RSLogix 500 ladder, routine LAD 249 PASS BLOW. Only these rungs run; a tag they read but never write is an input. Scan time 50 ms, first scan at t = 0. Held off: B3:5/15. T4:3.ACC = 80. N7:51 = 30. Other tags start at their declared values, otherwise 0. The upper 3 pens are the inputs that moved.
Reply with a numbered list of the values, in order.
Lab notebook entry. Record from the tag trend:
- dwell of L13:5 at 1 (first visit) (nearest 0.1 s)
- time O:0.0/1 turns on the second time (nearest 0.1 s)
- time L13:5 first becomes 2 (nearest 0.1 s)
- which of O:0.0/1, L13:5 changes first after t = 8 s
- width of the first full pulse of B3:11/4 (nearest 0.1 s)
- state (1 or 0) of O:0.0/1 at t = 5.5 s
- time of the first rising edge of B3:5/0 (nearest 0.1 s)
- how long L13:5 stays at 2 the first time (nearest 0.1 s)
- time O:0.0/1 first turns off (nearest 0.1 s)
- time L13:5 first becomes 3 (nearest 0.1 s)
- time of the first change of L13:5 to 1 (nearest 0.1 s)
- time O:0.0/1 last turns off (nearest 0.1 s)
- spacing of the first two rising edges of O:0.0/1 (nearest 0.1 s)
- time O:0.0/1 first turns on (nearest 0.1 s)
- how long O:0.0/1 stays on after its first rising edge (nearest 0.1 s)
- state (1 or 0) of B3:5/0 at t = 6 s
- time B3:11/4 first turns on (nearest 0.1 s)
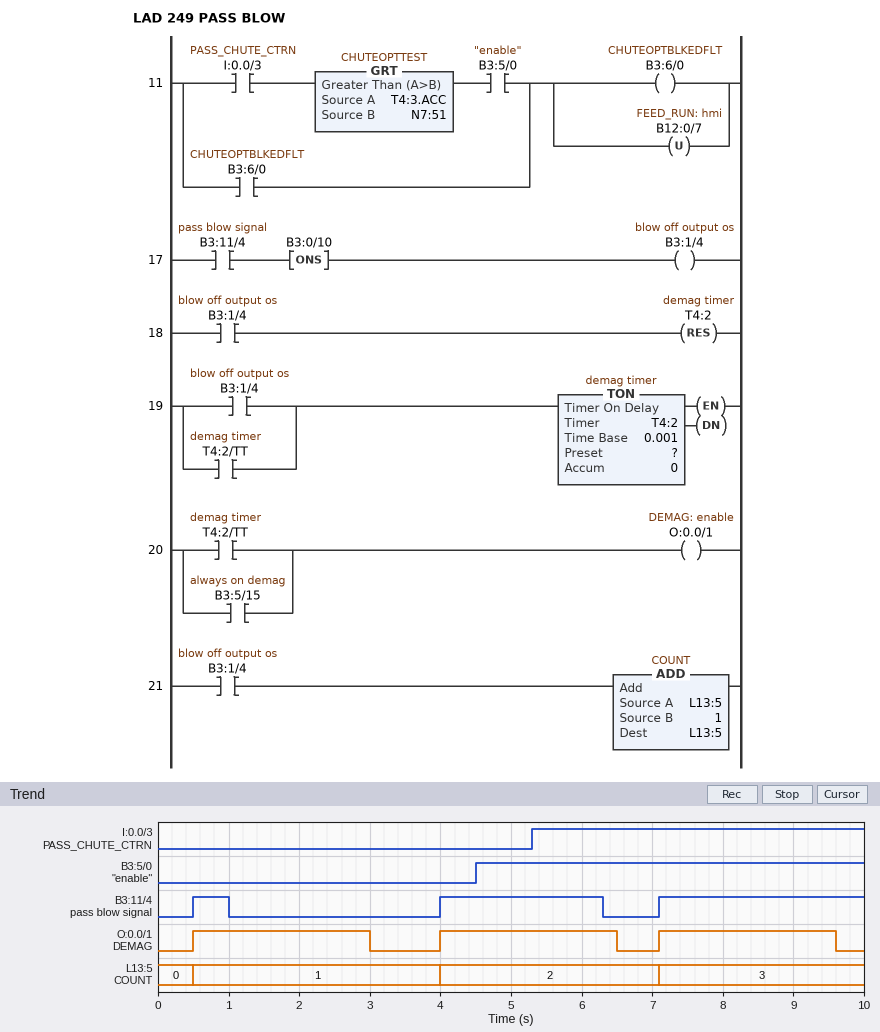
1. 3.5 s
2. 4.0 s
3. 4.0 s
4. O:0.0/1
5. 0.5 s
6. 1
7. 4.5 s
8. 3.1 s
9. 3.0 s
10. 7.1 s
11. 0.5 s
12. 9.6 s
13. 3.5 s
14. 0.5 s
15. 2.5 s
16. 1
17. 0.5 s
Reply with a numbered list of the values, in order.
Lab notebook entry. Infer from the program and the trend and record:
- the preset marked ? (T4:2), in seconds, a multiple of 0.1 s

1. 2.5 s
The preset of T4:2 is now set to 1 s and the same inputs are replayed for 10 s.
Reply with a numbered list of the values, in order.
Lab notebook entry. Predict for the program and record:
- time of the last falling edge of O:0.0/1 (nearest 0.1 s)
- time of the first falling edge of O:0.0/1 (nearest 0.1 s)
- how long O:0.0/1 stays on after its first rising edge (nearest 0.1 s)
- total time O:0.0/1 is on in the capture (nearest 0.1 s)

1. 8.1 s
2. 1.5 s
3. 1.0 s
4. 3.0 s
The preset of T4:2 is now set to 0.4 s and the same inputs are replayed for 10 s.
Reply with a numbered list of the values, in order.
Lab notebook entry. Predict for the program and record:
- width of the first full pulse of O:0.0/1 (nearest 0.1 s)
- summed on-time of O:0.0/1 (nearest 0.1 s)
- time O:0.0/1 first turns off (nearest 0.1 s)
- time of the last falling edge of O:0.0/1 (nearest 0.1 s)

1. 0.4 s
2. 1.2 s
3. 0.9 s
4. 7.5 s
